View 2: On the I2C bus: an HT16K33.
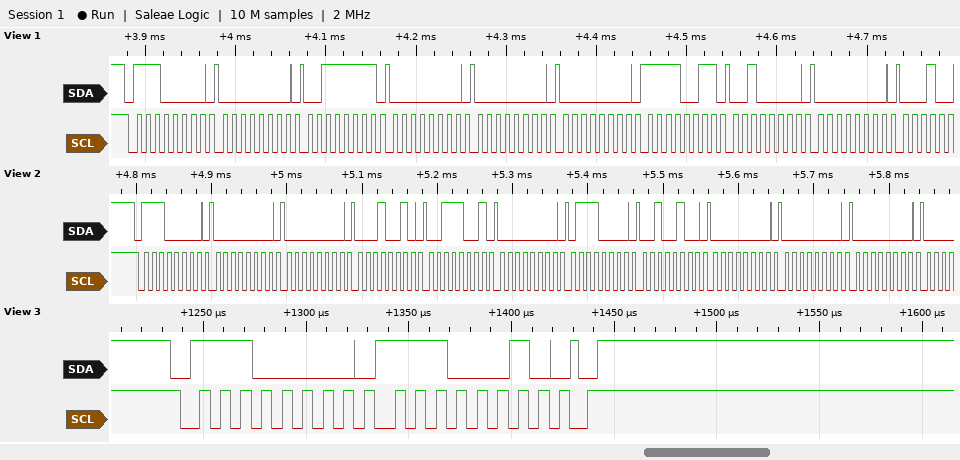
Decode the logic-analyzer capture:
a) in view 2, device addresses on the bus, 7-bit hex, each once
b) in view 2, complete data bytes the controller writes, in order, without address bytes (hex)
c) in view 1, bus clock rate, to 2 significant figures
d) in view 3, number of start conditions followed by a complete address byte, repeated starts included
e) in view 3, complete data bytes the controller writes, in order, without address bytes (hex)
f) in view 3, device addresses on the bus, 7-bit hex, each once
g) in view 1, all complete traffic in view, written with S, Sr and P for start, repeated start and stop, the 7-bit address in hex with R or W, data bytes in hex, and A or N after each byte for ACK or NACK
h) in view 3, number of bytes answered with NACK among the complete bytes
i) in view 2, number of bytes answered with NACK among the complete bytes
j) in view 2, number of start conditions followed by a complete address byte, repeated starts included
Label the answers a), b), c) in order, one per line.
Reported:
a) 0x70
b) 00 00 12 39 00 70 24 00 00 00
c) 100 kHz
d) 1
e) E2
f) 0x70
g) S 70W A 00 A 3F A 00 A 00 A 00 A F3 A 20 A 00 A
h) 0
i) 0
j) 1
